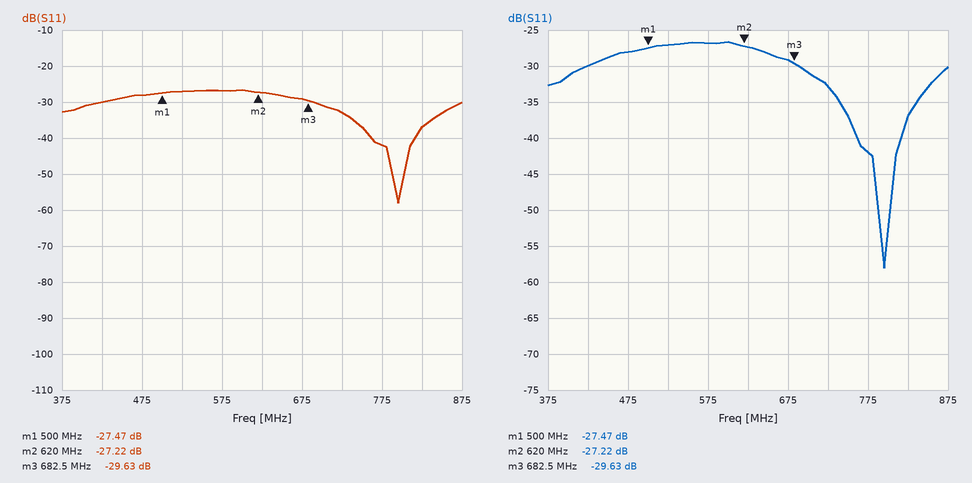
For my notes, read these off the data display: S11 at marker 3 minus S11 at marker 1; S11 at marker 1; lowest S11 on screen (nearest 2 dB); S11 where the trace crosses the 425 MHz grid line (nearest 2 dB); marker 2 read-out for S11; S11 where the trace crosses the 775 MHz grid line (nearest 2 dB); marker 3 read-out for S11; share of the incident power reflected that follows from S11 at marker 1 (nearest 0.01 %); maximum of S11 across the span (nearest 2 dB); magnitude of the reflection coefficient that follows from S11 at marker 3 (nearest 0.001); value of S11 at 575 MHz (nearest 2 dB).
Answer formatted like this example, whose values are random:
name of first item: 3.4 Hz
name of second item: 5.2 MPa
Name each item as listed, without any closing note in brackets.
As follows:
S11 at marker 3 minus S11 at marker 1: -2.16 dB
S11 at marker 1: -27.47 dB
lowest S11 on screen: -58 dB
S11 where the trace crosses the 425 MHz grid line: -30 dB
marker 2 read-out for S11: -27.22 dB
S11 where the trace crosses the 775 MHz grid line: -42 dB
marker 3 read-out for S11: -29.63 dB
share of the incident power reflected that follows from S11 at marker 1: 0.18 %
maximum of S11 across the span: -26 dB
magnitude of the reflection coefficient that follows from S11 at marker 3: 0.033
value of S11 at 575 MHz: -26 dB
